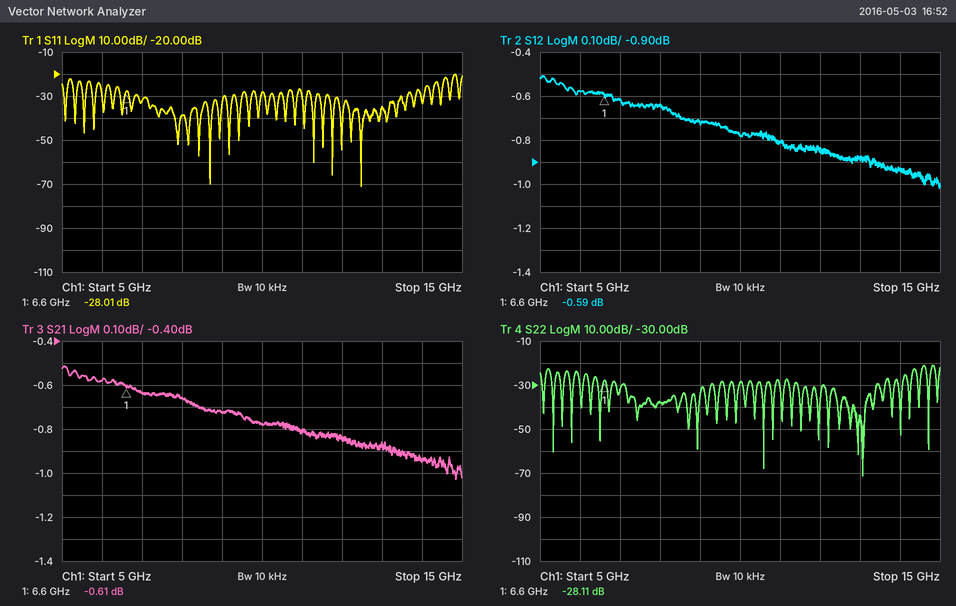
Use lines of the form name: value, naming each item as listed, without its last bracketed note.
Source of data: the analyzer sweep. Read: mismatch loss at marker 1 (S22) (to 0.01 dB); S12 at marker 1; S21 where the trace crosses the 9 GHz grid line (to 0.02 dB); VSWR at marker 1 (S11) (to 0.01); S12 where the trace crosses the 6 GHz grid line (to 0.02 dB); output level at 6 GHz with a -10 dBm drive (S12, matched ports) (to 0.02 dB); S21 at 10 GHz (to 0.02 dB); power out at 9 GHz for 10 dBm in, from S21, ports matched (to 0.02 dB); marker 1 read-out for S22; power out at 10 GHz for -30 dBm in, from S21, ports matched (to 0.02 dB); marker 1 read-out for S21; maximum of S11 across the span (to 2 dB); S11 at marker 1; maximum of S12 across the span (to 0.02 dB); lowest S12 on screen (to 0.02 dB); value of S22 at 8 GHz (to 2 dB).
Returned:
mismatch loss at marker 1 (S22): 0.01 dB
S12 at marker 1: -0.59 dB
S21 where the trace crosses the 9 GHz grid line: -0.72 dB
VSWR at marker 1 (S11): 1.08
S12 where the trace crosses the 6 GHz grid line: -0.58 dB
output level at 6 GHz with a -10 dBm drive (S12, matched ports): -10.58 dBm
S21 at 10 GHz: -0.78 dB
power out at 9 GHz for 10 dBm in, from S21, ports matched: 9.28 dBm
marker 1 read-out for S22: -28.11 dB
power out at 10 GHz for -30 dBm in, from S21, ports matched: -30.78 dBm
marker 1 read-out for S21: -0.61 dB
maximum of S11 across the span: -20 dB
S11 at marker 1: -28.01 dB
maximum of S12 across the span: -0.50 dB
lowest S12 on screen: -1.02 dB
value of S22 at 8 GHz: -38 dB
